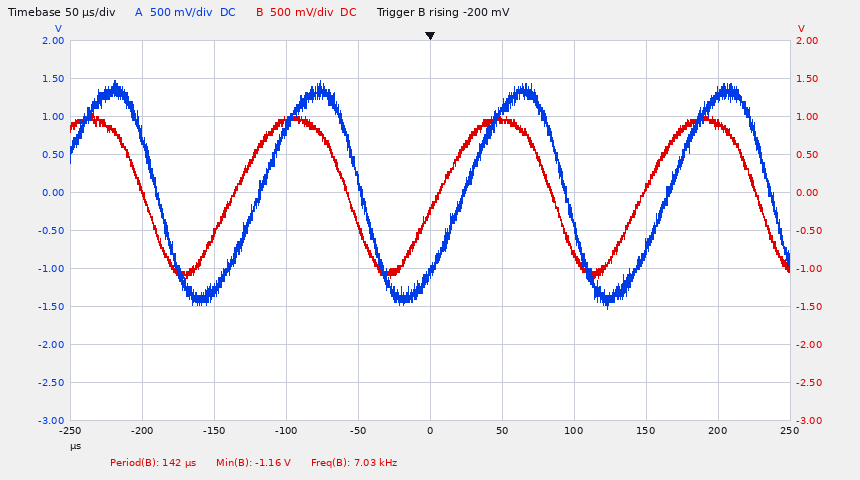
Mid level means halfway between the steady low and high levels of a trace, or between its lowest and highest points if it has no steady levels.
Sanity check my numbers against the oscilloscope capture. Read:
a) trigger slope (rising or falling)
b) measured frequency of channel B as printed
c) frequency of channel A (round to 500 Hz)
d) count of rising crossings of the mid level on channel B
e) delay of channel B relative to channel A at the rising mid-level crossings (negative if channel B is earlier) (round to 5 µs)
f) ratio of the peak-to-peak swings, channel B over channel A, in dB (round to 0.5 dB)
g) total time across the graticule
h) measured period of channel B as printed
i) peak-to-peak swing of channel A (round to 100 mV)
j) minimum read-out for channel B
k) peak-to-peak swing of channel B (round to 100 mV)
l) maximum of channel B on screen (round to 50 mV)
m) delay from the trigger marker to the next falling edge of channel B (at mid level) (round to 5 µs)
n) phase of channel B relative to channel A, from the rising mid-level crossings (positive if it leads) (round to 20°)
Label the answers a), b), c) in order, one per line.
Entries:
a) rising
b) 7.03 kHz
c) 7.0 kHz
d) 3
e) -20 µs
f) -2.5 dB
g) 500 µs
h) 142 µs
i) 3.00 V
j) -1.16 V
k) 2.20 V
l) 1.05 V
m) 85 µs
n) +40°
